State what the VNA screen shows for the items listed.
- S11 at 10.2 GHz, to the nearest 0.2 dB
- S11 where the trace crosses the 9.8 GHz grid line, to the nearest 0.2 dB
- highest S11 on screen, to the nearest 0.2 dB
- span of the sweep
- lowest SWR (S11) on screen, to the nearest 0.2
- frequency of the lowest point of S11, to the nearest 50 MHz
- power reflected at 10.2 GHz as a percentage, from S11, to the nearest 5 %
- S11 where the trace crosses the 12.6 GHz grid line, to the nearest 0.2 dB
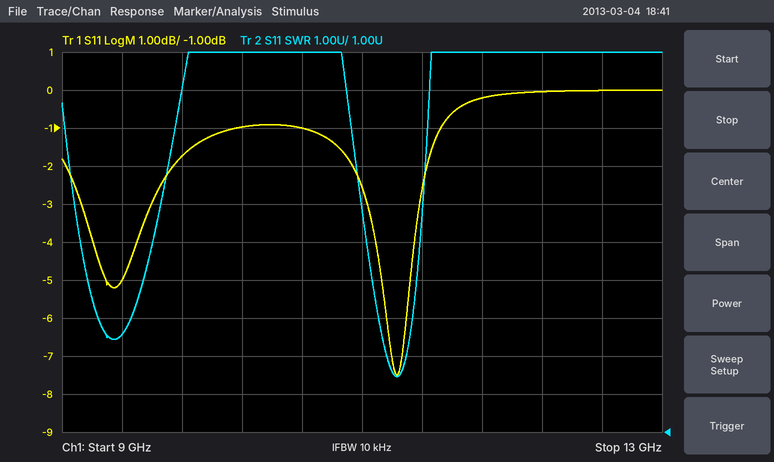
-1.0 dB
-1.8 dB
0.0 dB
4 GHz
2.4
11.25 GHz
80 %
0.0 dB
